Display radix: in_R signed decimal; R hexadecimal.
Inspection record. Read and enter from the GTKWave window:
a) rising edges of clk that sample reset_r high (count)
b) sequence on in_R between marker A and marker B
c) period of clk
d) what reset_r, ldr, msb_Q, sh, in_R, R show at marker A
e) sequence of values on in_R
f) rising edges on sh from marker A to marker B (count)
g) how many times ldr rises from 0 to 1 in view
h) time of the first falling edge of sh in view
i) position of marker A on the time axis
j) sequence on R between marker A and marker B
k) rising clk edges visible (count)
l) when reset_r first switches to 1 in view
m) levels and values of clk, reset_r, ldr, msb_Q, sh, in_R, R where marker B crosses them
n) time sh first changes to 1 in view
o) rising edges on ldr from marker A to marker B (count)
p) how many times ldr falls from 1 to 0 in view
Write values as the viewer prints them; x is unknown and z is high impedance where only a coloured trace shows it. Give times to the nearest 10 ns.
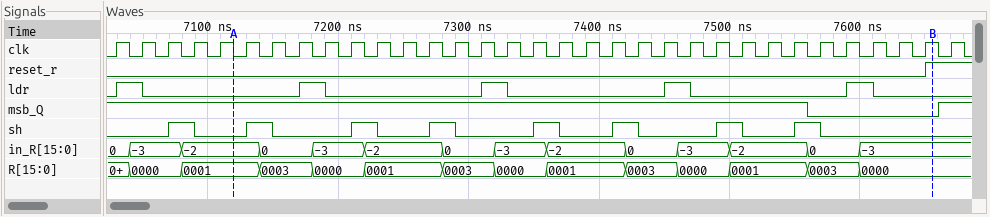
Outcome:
1
-2, 0, -3, -2, 0, -3, -2, 0, -3, -2, 0, -3
20 ns
reset_r=0, ldr=0, msb_Q=1, sh=0, in_R=-2, R=0001
0, -3, -2, 0, -3, -2, 0, -3, -2, 0, -3, -2, 0, -3
7
5
7090 ns
7120 ns
0001, 0003, 0000, 0001, 0003, 0000, 0001, 0003, 0000, 0001, 0003, 0000
33
7650 ns
clk=1, reset_r=1, ldr=0, msb_Q=0, sh=0, in_R=-3, R=0000
7070 ns
4
5
